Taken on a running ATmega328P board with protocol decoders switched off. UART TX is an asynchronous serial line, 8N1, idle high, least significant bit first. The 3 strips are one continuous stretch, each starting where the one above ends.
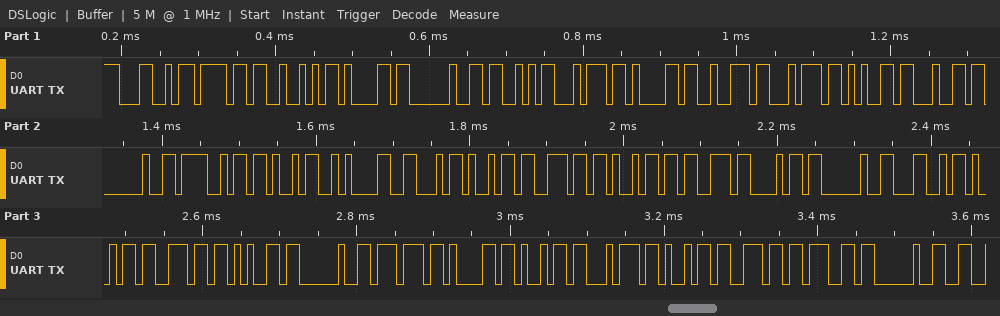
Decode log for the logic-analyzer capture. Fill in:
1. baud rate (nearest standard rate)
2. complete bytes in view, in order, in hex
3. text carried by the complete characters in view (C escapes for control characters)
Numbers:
115200 baud
4C 6F 52 61 20 53 74 61 72 74 65 64 20 4F 4B 0A 46 69 6E 69 73 68 20 4C 69 6E 65 20 77 61 69 74 69 6E 67 20
"LoRa Started OK\nFinish Line waiting "
